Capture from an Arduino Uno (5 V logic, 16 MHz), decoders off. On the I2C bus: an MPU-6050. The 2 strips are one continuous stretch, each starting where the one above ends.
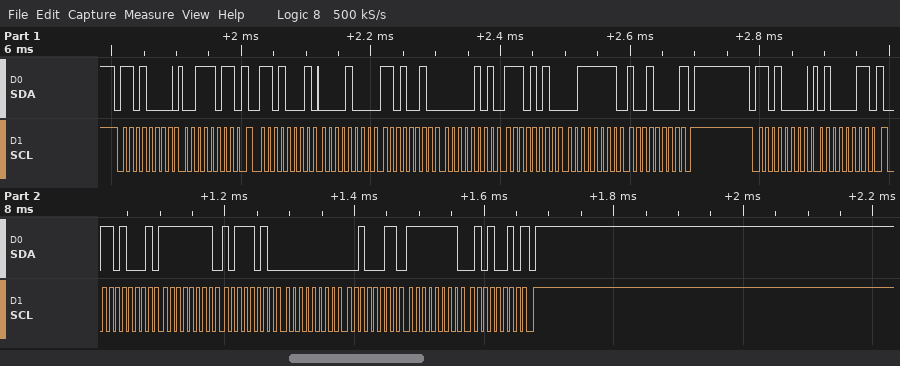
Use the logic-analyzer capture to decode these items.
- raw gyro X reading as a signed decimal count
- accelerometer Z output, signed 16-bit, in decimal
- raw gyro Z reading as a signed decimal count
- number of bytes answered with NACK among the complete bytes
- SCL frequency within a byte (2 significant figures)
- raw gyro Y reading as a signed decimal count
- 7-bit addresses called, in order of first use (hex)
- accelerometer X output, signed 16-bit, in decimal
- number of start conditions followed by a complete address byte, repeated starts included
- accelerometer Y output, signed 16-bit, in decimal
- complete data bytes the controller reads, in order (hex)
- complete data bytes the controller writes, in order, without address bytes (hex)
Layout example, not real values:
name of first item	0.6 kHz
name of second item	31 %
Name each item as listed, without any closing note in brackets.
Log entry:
raw gyro X reading as a signed decimal count	-70
accelerometer Z output, signed 16-bit, in decimal	16272
raw gyro Z reading as a signed decimal count	-174
number of bytes answered with NACK among the complete bytes	2
SCL frequency within a byte	100 kHz
raw gyro Y reading as a signed decimal count	35
7-bit addresses called, in order of first use	0x68
accelerometer X output, signed 16-bit, in decimal	2258
number of start conditions followed by a complete address byte, repeated starts included	4
accelerometer Y output, signed 16-bit, in decimal	1514
complete data bytes the controller reads, in order	08 D2 05 EA 3F 90 FF BA 00 23 FF 52
complete data bytes the controller writes, in order, without address bytes	3B 43
